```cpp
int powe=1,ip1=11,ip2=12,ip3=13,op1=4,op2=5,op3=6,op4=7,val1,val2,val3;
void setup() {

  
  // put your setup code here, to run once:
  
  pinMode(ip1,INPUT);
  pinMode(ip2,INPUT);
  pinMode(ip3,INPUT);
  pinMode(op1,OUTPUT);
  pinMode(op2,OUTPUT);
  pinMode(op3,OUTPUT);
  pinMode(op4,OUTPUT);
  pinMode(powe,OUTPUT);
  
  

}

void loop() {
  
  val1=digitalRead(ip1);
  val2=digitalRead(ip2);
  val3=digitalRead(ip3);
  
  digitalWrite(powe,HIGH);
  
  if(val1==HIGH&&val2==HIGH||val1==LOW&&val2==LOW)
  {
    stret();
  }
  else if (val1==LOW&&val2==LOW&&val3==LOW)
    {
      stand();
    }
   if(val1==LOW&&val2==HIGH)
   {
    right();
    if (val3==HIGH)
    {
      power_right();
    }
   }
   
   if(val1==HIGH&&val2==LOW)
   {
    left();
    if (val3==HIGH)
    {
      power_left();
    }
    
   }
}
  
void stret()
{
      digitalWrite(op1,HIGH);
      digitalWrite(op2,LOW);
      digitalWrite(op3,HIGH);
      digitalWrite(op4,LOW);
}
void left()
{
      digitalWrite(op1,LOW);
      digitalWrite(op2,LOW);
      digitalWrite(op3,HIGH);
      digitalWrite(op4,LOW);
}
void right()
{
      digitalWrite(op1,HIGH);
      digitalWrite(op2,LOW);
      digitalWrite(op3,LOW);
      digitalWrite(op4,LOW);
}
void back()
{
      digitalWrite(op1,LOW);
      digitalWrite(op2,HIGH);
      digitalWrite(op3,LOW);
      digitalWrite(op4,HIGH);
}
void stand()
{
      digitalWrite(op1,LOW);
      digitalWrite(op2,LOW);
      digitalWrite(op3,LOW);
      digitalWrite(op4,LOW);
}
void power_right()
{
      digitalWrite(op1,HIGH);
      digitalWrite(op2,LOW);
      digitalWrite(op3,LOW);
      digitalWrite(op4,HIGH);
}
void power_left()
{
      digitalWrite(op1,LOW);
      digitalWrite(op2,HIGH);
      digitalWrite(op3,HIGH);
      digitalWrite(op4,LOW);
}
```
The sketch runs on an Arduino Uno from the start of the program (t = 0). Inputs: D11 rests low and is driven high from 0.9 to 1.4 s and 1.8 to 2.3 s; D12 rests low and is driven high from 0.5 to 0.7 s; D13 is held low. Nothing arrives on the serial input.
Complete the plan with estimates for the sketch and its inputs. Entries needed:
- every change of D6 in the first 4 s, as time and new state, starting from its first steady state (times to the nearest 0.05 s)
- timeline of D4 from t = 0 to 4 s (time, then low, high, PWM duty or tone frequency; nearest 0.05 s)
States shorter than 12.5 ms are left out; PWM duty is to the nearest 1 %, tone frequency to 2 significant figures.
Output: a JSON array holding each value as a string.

["0 s high; 0.5 s low; 0.7 s high", "0 s high; 0.9 s low; 1.4 s high; 1.8 s low; 2.3 s high"]
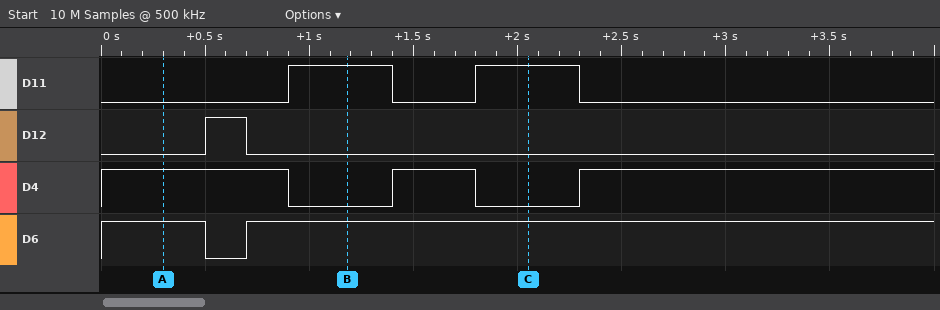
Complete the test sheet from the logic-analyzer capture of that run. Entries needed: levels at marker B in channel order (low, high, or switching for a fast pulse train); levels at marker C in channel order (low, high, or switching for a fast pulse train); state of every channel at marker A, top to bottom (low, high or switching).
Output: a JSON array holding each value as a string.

["D11 high, D12 low, D4 low, D6 high", "D11 high, D12 low, D4 low, D6 high", "D11 low, D12 low, D4 high, D6 high"]
